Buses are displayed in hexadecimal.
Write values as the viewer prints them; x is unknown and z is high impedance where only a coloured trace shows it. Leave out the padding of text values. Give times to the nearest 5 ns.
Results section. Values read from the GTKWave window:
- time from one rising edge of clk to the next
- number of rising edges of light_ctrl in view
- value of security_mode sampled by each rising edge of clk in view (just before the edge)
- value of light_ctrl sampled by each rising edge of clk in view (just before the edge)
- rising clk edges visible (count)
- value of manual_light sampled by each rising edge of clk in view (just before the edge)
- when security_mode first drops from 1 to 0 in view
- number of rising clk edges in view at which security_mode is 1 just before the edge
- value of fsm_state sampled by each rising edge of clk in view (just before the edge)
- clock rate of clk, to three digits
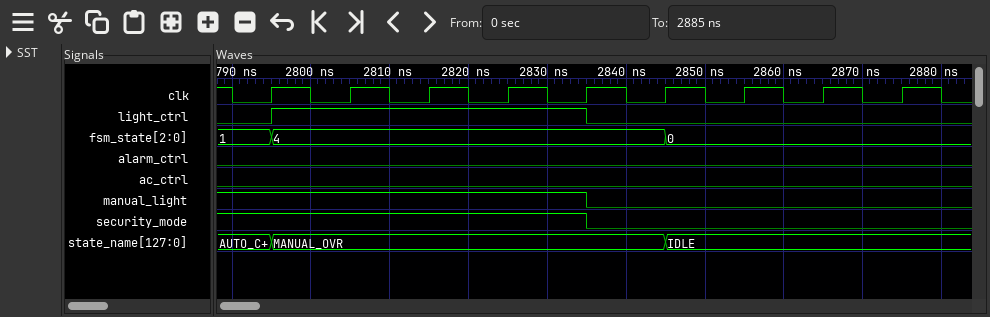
10 ns
1
1 1 1 1 1 0 0 0 0
0 1 1 1 1 0 0 0 0
9
1 1 1 1 1 0 0 0 0
2835 ns
5
1, 4, 4, 4, 4, 4, 0, 0, 0
100 MHz
